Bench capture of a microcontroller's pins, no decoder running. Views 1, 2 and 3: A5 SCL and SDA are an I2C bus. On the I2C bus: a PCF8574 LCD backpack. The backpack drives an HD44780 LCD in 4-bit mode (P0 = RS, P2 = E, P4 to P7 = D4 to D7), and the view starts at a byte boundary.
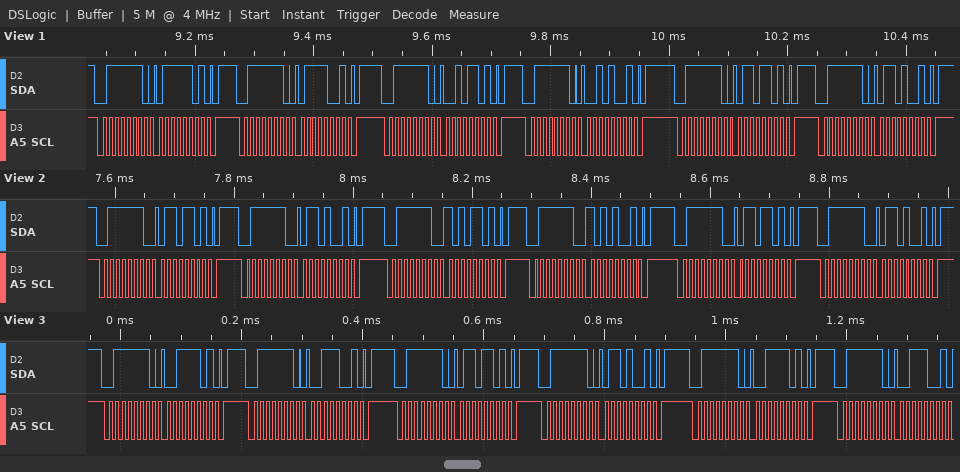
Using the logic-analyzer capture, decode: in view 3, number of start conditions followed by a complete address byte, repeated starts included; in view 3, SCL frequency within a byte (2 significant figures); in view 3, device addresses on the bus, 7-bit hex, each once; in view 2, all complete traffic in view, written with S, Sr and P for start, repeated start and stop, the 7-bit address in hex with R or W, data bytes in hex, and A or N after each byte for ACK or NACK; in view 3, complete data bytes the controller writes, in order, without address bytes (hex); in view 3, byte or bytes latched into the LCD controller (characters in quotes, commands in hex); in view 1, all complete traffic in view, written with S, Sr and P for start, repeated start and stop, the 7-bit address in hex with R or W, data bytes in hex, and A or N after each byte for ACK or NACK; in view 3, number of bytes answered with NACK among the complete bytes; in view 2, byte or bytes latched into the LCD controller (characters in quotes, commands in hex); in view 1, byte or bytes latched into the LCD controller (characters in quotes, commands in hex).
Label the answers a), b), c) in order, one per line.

a) 6
b) 100 kHz
c) 0x3F
d) S 3FW A 6D A P S 3FW A 69 A P S 3FW A AD A P S 3FW A A9 A P S 3FW A 6D A P S 3FW A 69 A P
e) 3D 39 6D 69 3D 39
f) '6'
g) S 3FW A 7D A P S 3FW A 79 A P S 3FW A 2D A P S 3FW A 29 A P S 3FW A 6D A P S 3FW A 69 A P
h) 0
i) 'j'
j) 'r'
